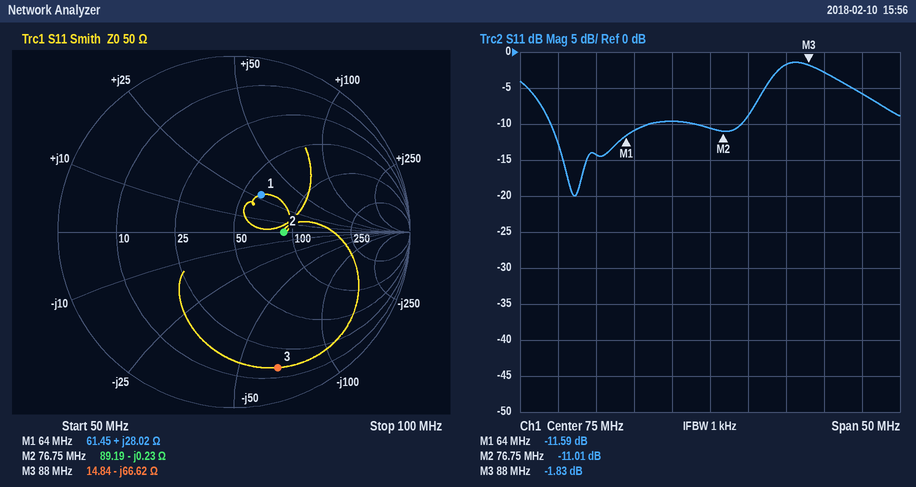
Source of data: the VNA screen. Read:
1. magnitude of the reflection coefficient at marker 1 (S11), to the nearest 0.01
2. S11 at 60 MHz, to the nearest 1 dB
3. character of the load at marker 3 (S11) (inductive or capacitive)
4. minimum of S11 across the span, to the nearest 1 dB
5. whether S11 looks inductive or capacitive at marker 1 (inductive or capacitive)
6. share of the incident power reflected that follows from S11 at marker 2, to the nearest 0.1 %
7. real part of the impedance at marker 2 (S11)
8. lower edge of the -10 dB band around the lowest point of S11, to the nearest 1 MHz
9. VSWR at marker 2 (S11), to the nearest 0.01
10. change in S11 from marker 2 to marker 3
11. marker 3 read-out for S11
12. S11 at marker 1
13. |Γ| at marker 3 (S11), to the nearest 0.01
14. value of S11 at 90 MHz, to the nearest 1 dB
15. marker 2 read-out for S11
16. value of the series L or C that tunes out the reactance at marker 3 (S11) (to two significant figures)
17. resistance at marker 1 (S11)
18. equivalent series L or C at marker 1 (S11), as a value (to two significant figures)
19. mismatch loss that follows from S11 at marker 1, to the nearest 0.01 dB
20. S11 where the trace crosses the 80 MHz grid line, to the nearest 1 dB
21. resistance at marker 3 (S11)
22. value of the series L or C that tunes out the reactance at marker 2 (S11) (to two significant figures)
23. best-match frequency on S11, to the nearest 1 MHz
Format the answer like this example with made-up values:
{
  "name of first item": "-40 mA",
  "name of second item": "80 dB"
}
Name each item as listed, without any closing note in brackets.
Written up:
{
  "magnitude of the reflection coefficient at marker 1 (S11), to the nearest 0.01": "0.26",
  "S11 at 60 MHz, to the nearest 1 dB": "-14 dB",
  "character of the load at marker 3 (S11)": "capacitive",
  "minimum of S11 across the span, to the nearest 1 dB": "-20 dB",
  "whether S11 looks inductive or capacitive at marker 1": "inductive",
  "share of the incident power reflected that follows from S11 at marker 2, to the nearest 0.1 %": "7.9 %",
  "real part of the impedance at marker 2": "89.19 Ω",
  "lower edge of the -10 dB band around the lowest point of S11, to the nearest 1 MHz": "54 MHz",
  "VSWR at marker 2 (S11), to the nearest 0.01": "1.78",
  "change in S11 from marker 2 to marker 3": "9.18 dB",
  "marker 3 read-out for S11": "-1.83 dB",
  "S11 at marker 1": "-11.59 dB",
  "|Γ| at marker 3 (S11), to the nearest 0.01": "0.81",
  "value of S11 at 90 MHz, to the nearest 1 dB": "-3 dB",
  "marker 2 read-out for S11": "-11.01 dB",
  "value of the series L or C that tunes out the reactance at marker 3 (S11)": "120 nH",
  "resistance at marker 1": "61.45 Ω",
  "equivalent series L or C at marker 1 (S11), as a value": "70 nH",
  "mismatch loss that follows from S11 at marker 1, to the nearest 0.01 dB": "0.31 dB",
  "S11 where the trace crosses the 80 MHz grid line, to the nearest 1 dB": "-9 dB",
  "resistance at marker 3": "14.84 Ω",
  "value of the series L or C that tunes out the reactance at marker 2 (S11)": "480 pH",
  "best-match frequency on S11, to the nearest 1 MHz": "57 MHz"
}
